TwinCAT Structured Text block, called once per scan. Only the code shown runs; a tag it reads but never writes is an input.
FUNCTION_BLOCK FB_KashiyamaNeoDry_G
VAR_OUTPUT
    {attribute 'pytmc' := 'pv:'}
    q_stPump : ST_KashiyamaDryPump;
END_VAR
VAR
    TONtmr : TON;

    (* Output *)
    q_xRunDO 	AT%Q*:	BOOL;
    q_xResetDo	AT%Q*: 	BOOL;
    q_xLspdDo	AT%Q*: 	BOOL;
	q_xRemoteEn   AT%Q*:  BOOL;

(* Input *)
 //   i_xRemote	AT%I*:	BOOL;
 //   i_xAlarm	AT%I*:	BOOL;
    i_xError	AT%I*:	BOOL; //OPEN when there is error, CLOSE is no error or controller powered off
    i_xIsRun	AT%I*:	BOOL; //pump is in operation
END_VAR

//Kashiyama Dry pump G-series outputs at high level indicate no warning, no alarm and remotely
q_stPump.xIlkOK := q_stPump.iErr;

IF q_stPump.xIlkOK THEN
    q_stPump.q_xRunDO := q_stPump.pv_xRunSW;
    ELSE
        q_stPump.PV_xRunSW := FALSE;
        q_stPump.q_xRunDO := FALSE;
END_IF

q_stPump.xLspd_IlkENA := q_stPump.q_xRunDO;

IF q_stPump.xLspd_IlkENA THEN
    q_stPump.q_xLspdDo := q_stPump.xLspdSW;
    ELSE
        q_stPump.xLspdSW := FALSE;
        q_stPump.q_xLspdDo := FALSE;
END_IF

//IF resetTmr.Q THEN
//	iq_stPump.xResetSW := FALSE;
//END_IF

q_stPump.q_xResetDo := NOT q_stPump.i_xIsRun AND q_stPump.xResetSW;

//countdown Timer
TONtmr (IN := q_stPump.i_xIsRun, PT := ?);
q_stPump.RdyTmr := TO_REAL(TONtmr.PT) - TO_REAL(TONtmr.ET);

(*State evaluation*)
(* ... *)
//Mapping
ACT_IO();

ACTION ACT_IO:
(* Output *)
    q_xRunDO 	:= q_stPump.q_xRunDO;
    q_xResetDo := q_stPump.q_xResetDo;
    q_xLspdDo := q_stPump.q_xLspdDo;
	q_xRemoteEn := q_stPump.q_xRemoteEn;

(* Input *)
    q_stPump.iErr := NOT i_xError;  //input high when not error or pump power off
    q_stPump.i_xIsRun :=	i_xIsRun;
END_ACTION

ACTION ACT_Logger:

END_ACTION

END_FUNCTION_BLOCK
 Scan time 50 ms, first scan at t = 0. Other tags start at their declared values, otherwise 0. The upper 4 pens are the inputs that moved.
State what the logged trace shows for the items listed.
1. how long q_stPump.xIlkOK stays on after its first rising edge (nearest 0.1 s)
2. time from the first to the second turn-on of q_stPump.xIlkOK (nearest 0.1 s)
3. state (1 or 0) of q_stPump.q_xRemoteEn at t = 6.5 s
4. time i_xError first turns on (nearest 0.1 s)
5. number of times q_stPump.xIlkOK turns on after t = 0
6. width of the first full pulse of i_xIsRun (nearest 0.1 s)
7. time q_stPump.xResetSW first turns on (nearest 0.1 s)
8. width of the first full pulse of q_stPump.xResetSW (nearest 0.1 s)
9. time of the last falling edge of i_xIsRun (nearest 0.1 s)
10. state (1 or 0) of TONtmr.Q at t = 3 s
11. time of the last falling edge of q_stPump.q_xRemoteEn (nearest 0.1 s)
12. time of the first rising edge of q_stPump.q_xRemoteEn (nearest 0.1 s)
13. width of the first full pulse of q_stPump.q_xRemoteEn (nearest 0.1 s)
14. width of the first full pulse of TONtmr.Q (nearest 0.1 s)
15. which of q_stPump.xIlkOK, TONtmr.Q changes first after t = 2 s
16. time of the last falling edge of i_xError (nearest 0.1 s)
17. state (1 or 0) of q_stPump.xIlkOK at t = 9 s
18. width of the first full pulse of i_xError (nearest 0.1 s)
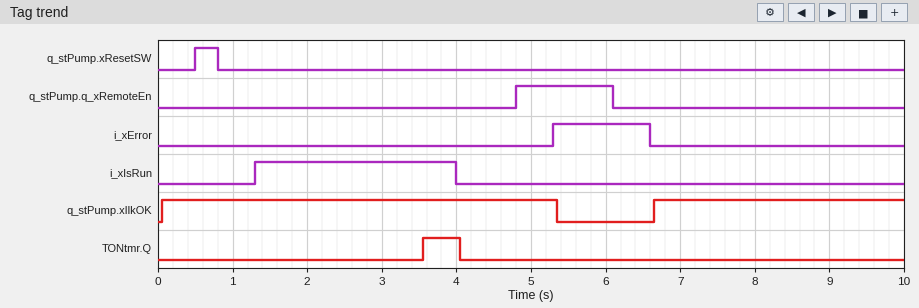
5.3 s
6.6 s
0
5.3 s
2
2.7 s
0.5 s
0.3 s
4.0 s
0
6.1 s
4.8 s
1.3 s
0.5 s
TONtmr.Q
6.6 s
1
1.3 s
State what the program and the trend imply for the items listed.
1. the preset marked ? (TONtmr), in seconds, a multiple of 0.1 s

2.2 s
